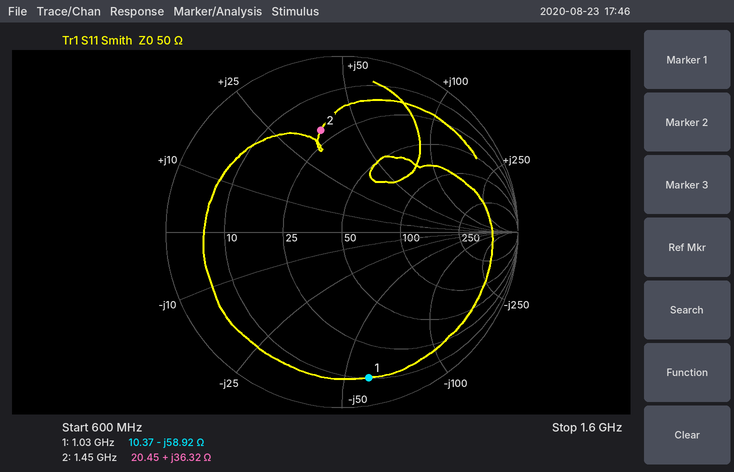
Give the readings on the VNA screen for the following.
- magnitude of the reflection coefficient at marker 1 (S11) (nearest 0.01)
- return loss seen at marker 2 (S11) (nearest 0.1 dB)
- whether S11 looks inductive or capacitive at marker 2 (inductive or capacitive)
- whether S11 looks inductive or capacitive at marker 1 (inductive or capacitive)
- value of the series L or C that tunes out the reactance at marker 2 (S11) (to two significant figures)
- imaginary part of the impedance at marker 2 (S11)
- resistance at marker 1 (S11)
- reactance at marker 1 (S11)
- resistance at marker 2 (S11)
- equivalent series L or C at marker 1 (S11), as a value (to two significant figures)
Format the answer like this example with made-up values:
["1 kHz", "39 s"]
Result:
["0.84", "4.6 dB", "inductive", "capacitive", "3.0 pF", "+36.32 Ω", "10.37 Ω", "-58.92 Ω", "20.45 Ω", "2.6 pF"]
